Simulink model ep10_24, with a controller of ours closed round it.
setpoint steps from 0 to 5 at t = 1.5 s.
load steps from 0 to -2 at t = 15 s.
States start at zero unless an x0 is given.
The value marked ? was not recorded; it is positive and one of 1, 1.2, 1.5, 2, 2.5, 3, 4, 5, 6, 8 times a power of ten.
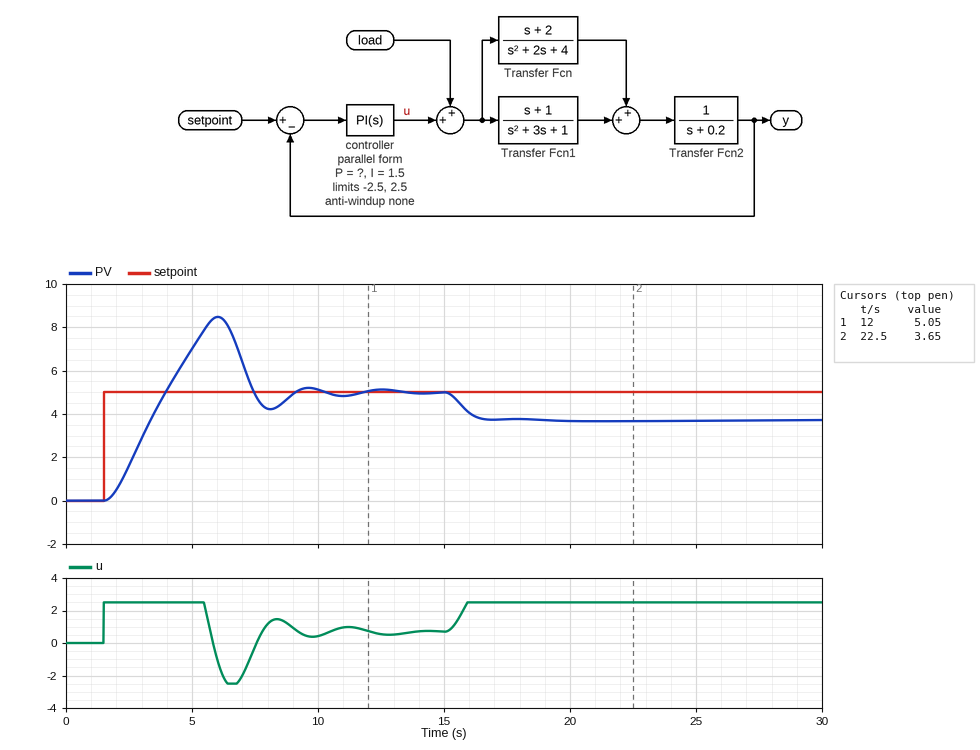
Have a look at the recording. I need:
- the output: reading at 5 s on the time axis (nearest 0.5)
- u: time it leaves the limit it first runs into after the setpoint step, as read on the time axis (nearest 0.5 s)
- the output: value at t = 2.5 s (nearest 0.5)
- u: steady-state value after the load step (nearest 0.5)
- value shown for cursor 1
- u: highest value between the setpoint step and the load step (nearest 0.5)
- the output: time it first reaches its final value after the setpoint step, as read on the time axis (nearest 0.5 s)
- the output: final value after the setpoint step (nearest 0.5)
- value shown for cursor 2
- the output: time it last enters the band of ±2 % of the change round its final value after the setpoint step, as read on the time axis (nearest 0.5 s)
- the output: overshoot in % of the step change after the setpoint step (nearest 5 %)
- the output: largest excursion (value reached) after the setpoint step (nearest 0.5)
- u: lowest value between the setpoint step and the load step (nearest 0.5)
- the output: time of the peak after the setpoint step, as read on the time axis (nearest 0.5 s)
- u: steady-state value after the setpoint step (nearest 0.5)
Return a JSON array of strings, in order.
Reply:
["7.0", "5.5 s", "1.5", "2.5", "5.05", "2.5", "4.0 s", "5.0", "3.65", "13.0 s", "70 %", "8.5", "-2.5", "6.0 s", "0.5"]
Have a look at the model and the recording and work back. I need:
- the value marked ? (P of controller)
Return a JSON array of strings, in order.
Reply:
["1.5"]
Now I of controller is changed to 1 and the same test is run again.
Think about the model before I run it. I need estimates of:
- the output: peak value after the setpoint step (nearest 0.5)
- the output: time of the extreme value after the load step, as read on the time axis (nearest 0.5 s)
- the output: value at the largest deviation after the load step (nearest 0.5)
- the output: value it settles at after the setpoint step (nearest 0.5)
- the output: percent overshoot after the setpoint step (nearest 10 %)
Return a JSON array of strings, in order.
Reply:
["8.0", "20.5 s", "3.5", "5.0", "60 %"]
